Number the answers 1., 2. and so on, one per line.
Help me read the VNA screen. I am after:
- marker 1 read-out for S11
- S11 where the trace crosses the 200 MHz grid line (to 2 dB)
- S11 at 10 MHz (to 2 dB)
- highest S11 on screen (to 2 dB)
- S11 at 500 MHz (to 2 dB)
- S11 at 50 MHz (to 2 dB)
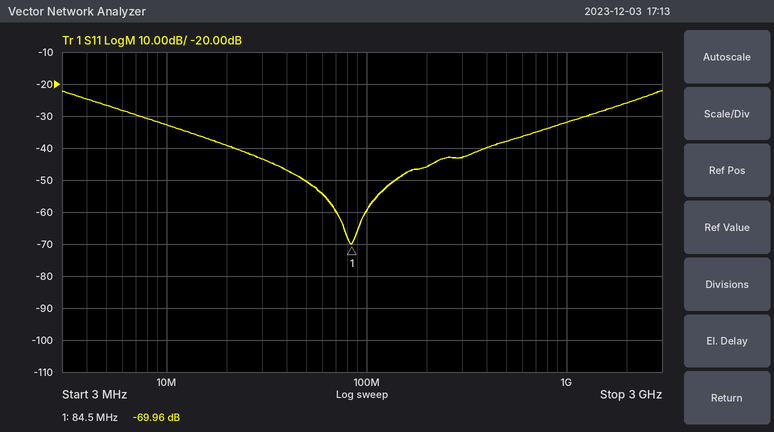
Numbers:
1. -69.96 dB
2. -46 dB
3. -32 dB
4. -22 dB
5. -38 dB
6. -50 dB
